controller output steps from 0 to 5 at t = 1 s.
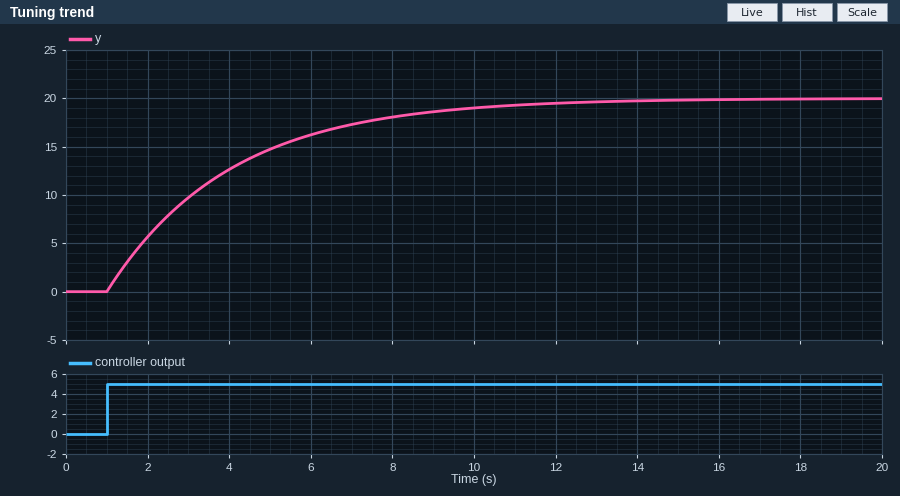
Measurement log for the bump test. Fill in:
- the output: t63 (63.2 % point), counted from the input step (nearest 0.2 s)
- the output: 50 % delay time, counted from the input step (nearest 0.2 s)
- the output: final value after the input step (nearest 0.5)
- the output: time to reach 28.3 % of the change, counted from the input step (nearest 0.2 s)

3.0 s
2.0 s
20.0
1.0 s
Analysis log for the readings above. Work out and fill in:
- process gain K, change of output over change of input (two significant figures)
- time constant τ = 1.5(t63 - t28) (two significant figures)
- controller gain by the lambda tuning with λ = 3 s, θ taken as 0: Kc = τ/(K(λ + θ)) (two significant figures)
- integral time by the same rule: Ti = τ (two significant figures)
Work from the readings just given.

4.0
3.0 s
0.25
3.0 s
